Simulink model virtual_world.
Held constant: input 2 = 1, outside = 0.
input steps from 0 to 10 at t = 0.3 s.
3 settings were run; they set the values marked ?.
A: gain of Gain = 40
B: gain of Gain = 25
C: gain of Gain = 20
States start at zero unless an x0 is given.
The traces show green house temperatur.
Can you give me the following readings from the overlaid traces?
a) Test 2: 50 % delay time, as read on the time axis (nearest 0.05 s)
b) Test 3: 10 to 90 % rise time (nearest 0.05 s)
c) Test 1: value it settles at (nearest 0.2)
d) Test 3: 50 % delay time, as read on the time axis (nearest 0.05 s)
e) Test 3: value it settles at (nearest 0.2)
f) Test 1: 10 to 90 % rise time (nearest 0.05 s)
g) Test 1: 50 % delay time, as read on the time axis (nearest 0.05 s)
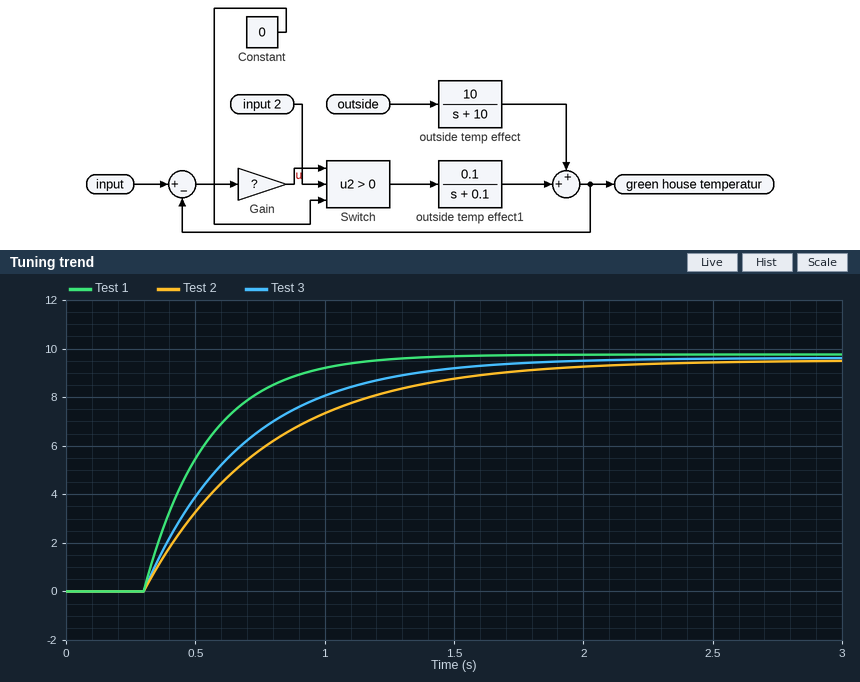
0.65 s
0.85 s
9.8
0.55 s
9.6
0.55 s
0.45 s
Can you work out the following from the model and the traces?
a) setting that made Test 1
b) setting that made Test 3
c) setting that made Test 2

A
B
C
